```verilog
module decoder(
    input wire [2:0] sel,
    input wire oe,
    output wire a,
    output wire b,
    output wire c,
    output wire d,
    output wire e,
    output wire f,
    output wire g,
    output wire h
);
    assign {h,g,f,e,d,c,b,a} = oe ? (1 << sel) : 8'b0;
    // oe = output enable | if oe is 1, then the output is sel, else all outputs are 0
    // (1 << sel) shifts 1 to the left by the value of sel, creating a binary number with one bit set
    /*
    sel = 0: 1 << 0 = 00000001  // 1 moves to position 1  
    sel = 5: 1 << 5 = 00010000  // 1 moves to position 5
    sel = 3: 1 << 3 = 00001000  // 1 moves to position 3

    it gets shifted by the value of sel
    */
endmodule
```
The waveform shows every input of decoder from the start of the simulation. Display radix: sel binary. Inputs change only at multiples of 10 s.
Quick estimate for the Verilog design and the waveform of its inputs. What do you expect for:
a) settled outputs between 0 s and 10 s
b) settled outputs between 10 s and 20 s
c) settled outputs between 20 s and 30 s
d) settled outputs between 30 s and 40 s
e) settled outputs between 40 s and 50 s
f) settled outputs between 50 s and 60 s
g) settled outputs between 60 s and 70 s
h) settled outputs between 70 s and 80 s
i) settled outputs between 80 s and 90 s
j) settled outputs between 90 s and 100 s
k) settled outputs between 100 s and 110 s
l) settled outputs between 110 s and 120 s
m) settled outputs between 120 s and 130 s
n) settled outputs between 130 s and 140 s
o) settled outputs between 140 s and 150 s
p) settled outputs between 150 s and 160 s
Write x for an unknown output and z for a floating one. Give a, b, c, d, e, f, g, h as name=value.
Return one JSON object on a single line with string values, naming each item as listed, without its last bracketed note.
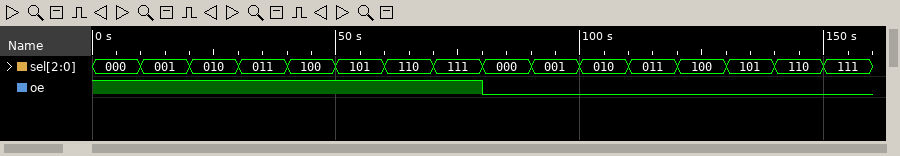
{"settled outputs between 0 s and 10 s": "a=1, b=0, c=0, d=0, e=0, f=0, g=0, h=0", "settled outputs between 10 s and 20 s": "a=0, b=1, c=0, d=0, e=0, f=0, g=0, h=0", "settled outputs between 20 s and 30 s": "a=0, b=0, c=1, d=0, e=0, f=0, g=0, h=0", "settled outputs between 30 s and 40 s": "a=0, b=0, c=0, d=1, e=0, f=0, g=0, h=0", "settled outputs between 40 s and 50 s": "a=0, b=0, c=0, d=0, e=1, f=0, g=0, h=0", "settled outputs between 50 s and 60 s": "a=0, b=0, c=0, d=0, e=0, f=1, g=0, h=0", "settled outputs between 60 s and 70 s": "a=0, b=0, c=0, d=0, e=0, f=0, g=1, h=0", "settled outputs between 70 s and 80 s": "a=0, b=0, c=0, d=0, e=0, f=0, g=0, h=1", "settled outputs between 80 s and 90 s": "a=0, b=0, c=0, d=0, e=0, f=0, g=0, h=0", "settled outputs between 90 s and 100 s": "a=0, b=0, c=0, d=0, e=0, f=0, g=0, h=0", "settled outputs between 100 s and 110 s": "a=0, b=0, c=0, d=0, e=0, f=0, g=0, h=0", "settled outputs between 110 s and 120 s": "a=0, b=0, c=0, d=0, e=0, f=0, g=0, h=0", "settled outputs between 120 s and 130 s": "a=0, b=0, c=0, d=0, e=0, f=0, g=0, h=0", "settled outputs between 130 s and 140 s": "a=0, b=0, c=0, d=0, e=0, f=0, g=0, h=0", "settled outputs between 140 s and 150 s": "a=0, b=0, c=0, d=0, e=0, f=0, g=0, h=0", "settled outputs between 150 s and 160 s": "a=0, b=0, c=0, d=0, e=0, f=0, g=0, h=0"}
